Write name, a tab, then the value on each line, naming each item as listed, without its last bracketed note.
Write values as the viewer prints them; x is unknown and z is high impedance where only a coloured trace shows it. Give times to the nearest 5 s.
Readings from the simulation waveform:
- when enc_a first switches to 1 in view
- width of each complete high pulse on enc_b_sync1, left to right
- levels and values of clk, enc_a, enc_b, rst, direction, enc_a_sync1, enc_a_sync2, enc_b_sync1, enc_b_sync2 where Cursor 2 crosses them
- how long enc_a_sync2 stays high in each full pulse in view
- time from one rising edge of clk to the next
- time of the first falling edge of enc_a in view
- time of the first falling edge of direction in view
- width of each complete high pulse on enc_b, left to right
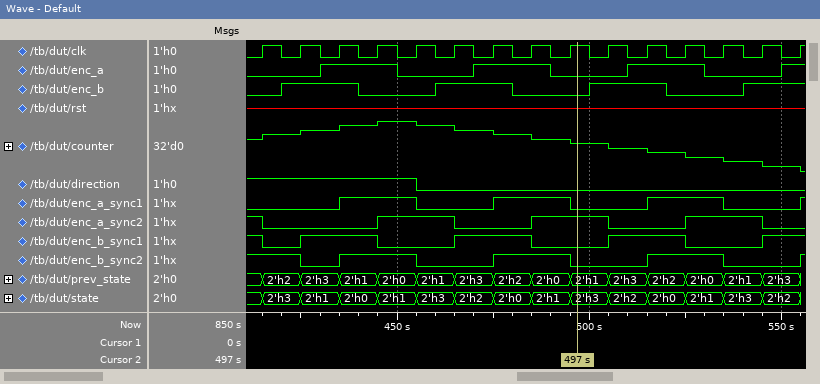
when enc_a first switches to 1 in view	430 s
width of each complete high pulse on enc_b_sync1, left to right	20 s, 20 s, 20 s
levels and values of clk, enc_a, enc_b, rst, direction, enc_a_sync1, enc_a_sync2, enc_b_sync1, enc_b_sync2 where Cursor 2 crosses them	clk=1, enc_a=0, enc_b=0, rst=x, direction=0, enc_a_sync1=0, enc_a_sync2=1, enc_b_sync1=0, enc_b_sync2=0
how long enc_a_sync2 stays high in each full pulse in view	20 s, 20 s, 20 s
time from one rising edge of clk to the next	10 s
time of the first falling edge of enc_a in view	450 s
time of the first falling edge of direction in view	455 s
width of each complete high pulse on enc_b, left to right	20 s, 20 s, 20 s
